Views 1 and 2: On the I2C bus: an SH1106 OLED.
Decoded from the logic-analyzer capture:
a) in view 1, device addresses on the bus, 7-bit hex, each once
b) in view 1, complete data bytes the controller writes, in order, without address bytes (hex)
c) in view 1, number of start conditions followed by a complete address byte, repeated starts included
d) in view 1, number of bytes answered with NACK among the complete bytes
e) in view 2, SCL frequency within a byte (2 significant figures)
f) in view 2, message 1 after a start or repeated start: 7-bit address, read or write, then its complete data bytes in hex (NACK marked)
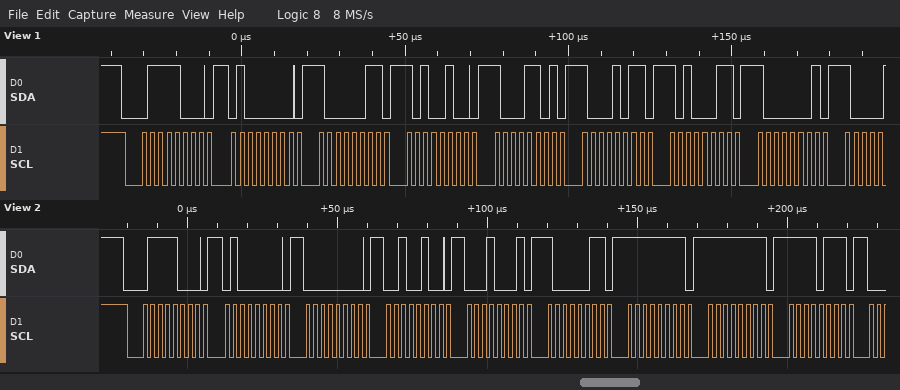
0x3C
40 83 A4 8D 8B A3 81
1
0
400 kHz
0x3C write: 40 00 24 11 83 FF FF F7
